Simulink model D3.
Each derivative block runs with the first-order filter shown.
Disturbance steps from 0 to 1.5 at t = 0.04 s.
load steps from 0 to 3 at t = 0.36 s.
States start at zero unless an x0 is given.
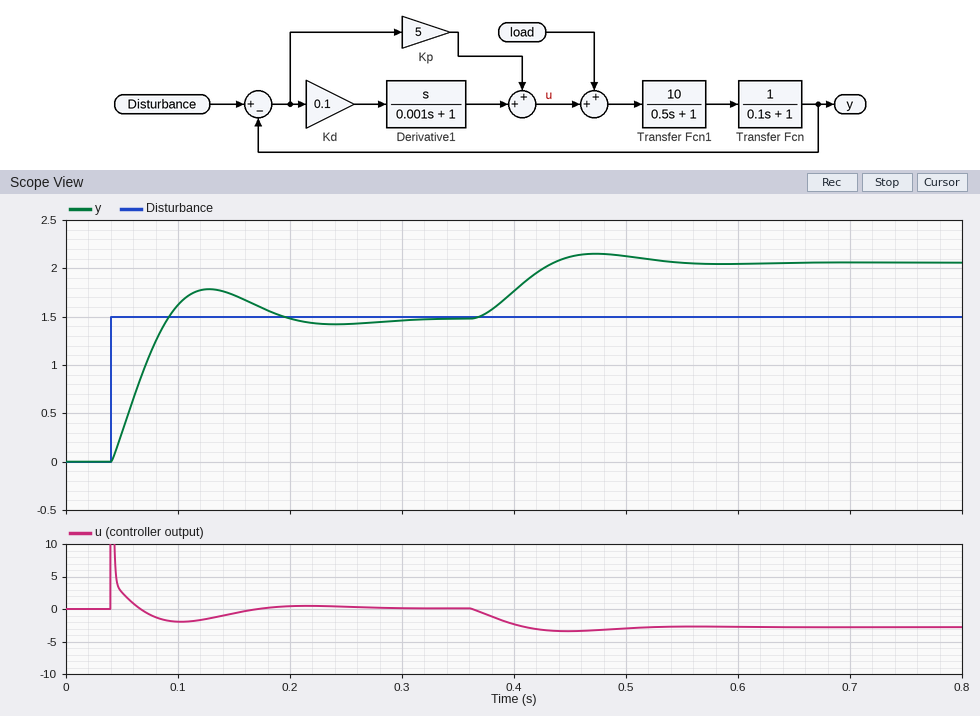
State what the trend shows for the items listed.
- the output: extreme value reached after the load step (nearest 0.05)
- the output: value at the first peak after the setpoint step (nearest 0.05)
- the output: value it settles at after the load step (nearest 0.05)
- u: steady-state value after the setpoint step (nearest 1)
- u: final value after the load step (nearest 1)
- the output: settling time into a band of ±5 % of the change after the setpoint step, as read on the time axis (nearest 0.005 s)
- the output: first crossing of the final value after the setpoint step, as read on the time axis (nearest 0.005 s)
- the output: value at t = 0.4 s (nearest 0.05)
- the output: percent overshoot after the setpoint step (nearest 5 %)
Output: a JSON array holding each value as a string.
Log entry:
["2.15", "1.80", "2.05", "0", "-3", "0.185 s", "0.090 s", "1.75", "20 %"]
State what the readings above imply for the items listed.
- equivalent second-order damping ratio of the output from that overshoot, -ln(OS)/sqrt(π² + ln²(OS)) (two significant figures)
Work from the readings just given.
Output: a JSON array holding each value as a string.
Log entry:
["0.46"]
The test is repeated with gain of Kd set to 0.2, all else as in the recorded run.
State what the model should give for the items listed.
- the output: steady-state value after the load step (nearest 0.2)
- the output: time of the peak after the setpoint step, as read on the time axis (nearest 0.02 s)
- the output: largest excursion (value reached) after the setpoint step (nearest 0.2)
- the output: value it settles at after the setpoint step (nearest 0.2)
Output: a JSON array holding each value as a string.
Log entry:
["2.0", "0.12 s", "1.6", "1.4"]
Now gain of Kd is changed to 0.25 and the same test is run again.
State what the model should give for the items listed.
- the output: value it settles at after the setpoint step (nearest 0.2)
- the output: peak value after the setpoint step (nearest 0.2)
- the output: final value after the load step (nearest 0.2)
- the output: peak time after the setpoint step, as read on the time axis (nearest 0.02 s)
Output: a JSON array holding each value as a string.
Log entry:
["1.4", "1.6", "2.0", "0.12 s"]
